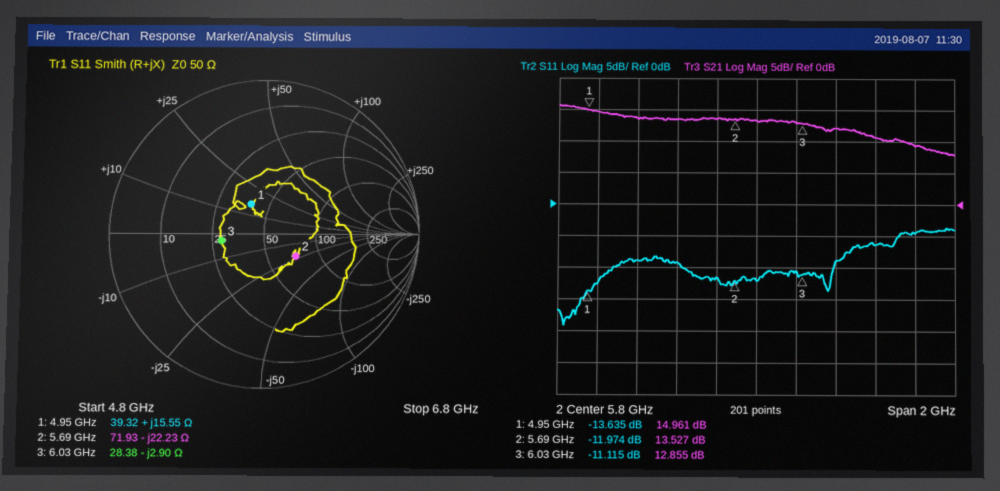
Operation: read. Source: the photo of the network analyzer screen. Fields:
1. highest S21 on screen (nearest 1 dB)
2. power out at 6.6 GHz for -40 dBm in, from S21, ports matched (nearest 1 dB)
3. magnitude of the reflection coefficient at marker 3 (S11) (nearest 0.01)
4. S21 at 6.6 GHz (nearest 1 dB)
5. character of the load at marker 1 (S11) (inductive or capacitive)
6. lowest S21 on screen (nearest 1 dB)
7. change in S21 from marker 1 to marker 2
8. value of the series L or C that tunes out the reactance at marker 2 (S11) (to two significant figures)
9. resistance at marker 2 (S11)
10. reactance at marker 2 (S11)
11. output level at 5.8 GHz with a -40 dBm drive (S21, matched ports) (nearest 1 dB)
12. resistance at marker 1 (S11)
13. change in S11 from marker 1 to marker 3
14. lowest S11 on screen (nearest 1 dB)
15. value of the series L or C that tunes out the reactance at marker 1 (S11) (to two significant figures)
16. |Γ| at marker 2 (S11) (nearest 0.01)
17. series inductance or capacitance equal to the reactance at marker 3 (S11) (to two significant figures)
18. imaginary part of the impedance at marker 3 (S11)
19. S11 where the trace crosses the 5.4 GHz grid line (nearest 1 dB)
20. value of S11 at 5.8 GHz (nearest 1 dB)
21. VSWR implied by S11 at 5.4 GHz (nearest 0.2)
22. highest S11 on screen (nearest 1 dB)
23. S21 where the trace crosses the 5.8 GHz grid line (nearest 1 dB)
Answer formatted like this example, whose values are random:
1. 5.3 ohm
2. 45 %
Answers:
1. 16 dB
2. -31 dBm
3. 0.28
4. 9 dB
5. inductive
6. 8 dB
7. -1.434 dB
8. 620 pH
9. 71.93 Ω
10. -22.23 Ω
11. -27 dBm
12. 39.32 Ω
13. 2.520 dB
14. -19 dB
15. 2.1 pF
16. 0.25
17. 9.1 pF
18. -2.90 Ω
19. -9 dB
20. -12 dB
21. 2.0
22. -4 dB
23. 13 dB
